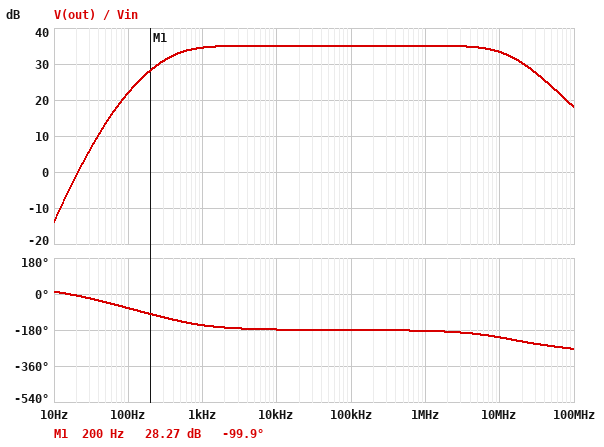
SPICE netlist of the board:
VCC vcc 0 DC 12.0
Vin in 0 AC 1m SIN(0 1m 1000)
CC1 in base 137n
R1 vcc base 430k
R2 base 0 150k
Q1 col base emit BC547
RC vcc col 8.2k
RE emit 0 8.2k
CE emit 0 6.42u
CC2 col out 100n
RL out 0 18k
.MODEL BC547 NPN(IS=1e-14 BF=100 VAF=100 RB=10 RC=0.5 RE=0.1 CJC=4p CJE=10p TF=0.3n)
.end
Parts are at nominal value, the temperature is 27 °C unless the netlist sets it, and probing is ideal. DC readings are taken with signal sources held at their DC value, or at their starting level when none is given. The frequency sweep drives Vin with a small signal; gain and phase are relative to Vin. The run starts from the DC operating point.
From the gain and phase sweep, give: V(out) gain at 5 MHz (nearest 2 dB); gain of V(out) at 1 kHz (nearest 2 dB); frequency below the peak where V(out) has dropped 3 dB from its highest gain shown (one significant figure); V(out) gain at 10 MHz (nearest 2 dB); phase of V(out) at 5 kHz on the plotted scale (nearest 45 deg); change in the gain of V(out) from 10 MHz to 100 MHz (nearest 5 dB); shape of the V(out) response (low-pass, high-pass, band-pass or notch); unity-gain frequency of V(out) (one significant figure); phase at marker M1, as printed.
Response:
34 dB
34 dB
400 Hz
34 dB
-180 deg
-15 dB
band-pass
20 Hz
-99.9 deg
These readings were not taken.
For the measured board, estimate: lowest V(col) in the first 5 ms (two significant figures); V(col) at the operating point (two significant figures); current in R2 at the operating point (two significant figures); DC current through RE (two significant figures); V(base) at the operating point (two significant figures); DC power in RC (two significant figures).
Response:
9.8 V
9.8 V
19 µA
270 µA
2.8 V
580 µW
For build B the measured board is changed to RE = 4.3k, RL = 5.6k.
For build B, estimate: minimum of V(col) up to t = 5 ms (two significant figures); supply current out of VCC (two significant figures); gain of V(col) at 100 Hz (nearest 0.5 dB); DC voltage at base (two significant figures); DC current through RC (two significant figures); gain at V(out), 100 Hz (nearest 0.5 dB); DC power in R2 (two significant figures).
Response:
8.2 V
480 µA
25.0 dB
2.6 V
460 µA
15.5 dB
46 µW
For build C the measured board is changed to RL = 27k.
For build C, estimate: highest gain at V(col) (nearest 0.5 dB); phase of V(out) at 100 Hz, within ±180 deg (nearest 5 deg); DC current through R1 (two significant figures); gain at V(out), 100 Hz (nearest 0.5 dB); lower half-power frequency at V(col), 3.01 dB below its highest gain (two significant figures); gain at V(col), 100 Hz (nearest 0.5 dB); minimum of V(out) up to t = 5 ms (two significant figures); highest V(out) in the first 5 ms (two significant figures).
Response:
36.0 dB
-80 deg
21 µA
23.5 dB
370 Hz
25.0 dB
-60 mV
63 mV
